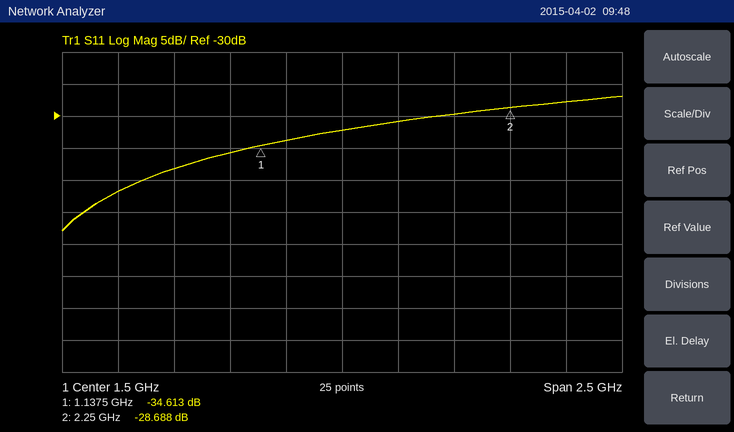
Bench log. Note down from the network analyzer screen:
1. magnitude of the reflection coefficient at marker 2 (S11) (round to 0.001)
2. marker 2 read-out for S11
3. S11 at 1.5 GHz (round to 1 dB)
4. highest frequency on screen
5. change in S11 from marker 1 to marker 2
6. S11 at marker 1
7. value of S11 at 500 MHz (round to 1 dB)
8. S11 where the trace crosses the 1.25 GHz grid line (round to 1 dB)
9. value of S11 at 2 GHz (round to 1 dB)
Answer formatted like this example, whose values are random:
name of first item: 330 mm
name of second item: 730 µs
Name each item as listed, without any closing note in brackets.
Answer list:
magnitude of the reflection coefficient at marker 2 (S11): 0.037
marker 2 read-out for S11: -28.688 dB
S11 at 1.5 GHz: -32 dB
highest frequency on screen: 2.75 GHz
change in S11 from marker 1 to marker 2: 5.925 dB
S11 at marker 1: -34.613 dB
value of S11 at 500 MHz: -42 dB
S11 where the trace crosses the 1.25 GHz grid line: -34 dB
value of S11 at 2 GHz: -30 dB
